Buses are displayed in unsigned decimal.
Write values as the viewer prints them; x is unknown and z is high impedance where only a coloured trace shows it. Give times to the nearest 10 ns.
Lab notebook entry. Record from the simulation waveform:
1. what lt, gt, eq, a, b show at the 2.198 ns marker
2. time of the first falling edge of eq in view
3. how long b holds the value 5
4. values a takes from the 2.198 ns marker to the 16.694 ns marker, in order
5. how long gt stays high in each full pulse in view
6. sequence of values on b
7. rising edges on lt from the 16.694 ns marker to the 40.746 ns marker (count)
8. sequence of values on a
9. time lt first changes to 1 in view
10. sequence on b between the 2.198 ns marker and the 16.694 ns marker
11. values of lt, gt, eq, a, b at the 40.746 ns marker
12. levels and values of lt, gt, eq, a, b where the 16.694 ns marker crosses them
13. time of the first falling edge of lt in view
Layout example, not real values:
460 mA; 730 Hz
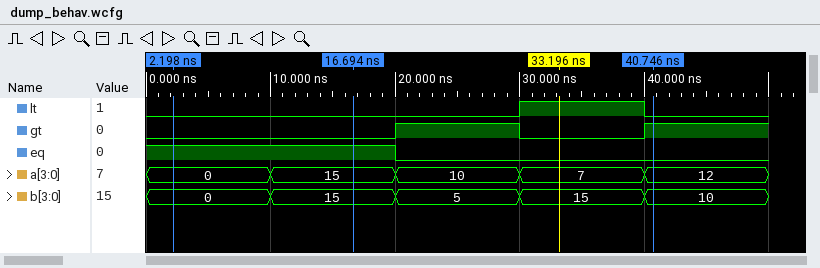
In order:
lt=0, gt=0, eq=1, a=0, b=0; 20 ns; 10 ns; 0, 15; 10 ns; 0, 15, 5, 15, 10; 1; 0, 15, 10, 7, 12; 30 ns; 0, 15; lt=0, gt=1, eq=0, a=12, b=10; lt=0, gt=0, eq=1, a=15, b=15; 40 ns
